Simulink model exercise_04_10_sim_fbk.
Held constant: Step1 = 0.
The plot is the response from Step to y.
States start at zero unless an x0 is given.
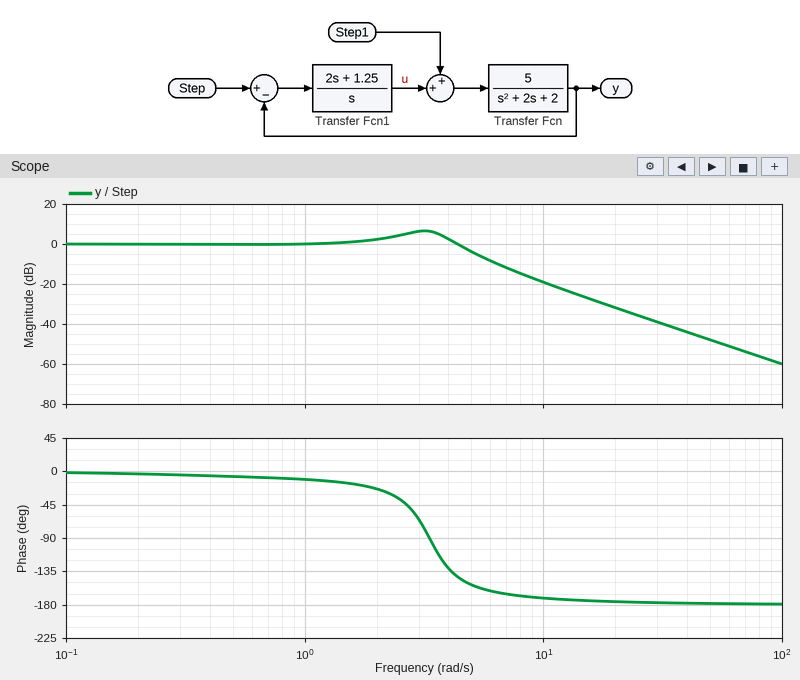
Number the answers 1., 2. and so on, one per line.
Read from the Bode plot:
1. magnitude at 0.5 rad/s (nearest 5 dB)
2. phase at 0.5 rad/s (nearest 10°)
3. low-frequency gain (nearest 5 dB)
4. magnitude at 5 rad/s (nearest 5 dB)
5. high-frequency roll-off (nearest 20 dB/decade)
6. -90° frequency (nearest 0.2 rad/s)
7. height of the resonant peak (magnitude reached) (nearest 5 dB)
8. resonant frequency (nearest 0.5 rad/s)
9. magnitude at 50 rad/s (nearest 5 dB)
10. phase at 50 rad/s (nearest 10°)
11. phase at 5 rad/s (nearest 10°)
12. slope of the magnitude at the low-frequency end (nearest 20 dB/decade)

1. 0 dB
2. -10°
3. 0 dB
4. -5 dB
5. -40 dB/decade
6. 3.4 rad/s
7. 5 dB
8. 3.0 rad/s
9. -50 dB
10. -180°
11. -150°
12. 0 dB/decade
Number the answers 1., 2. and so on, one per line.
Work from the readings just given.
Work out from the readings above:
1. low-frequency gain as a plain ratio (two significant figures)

1. 1.0
